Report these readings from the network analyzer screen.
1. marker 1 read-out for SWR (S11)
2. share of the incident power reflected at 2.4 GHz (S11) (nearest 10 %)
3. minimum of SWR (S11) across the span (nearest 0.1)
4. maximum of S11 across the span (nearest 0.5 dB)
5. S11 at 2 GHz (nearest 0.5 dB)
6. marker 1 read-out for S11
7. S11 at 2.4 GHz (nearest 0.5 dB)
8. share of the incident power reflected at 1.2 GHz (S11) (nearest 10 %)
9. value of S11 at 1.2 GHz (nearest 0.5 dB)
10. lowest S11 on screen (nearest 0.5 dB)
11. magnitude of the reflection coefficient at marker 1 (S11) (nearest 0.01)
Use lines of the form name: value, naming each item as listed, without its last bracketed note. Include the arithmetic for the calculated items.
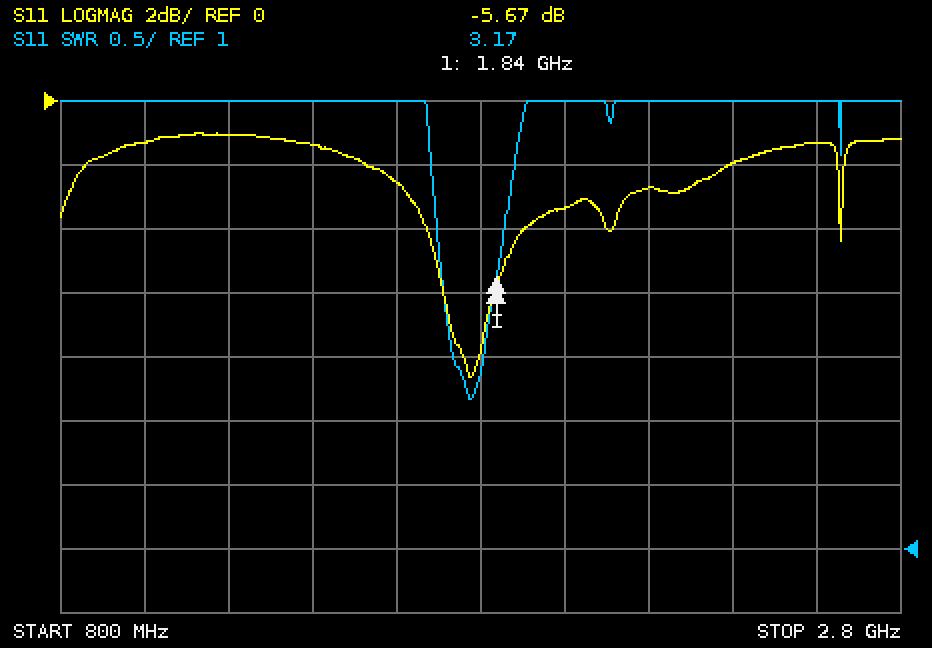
marker 1 read-out for SWR: 3.17
share of the incident power reflected at 2.4 GHz (S11): 10^(-2/10) ≈ 63.1 %, so 60 % to the nearest 10 %
minimum of SWR (S11) across the span: 2.2
maximum of S11 across the span: -1.0 dB
S11 at 2 GHz: -3.5 dB
marker 1 read-out for S11: -5.67 dB
S11 at 2.4 GHz: -2.0 dB
share of the incident power reflected at 1.2 GHz (S11): 10^(-1/10) ≈ 79.4 %, so 80 % to the nearest 10 %
value of S11 at 1.2 GHz: -1.0 dB
lowest S11 on screen: -8.5 dB
magnitude of the reflection coefficient at marker 1 (S11): 10^(-5.67/20) ≈ 0.52
